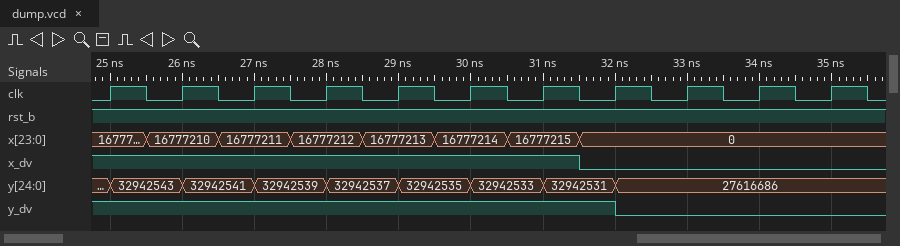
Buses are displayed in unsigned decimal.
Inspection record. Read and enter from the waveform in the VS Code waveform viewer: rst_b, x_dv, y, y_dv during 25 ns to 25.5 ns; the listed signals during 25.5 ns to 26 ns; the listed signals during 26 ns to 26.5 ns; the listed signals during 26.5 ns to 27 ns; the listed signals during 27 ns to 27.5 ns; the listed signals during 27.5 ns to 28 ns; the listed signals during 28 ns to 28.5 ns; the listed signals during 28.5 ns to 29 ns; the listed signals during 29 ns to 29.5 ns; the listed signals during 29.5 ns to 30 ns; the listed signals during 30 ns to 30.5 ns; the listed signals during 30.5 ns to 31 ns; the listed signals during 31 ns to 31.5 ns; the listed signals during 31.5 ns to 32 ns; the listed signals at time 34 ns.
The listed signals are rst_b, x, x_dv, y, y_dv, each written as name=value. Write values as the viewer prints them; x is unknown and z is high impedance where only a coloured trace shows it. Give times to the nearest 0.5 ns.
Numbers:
rst_b=1, x_dv=1, y=32942543, y_dv=1
rst_b=1, x=16777210, x_dv=1, y=32942543, y_dv=1
rst_b=1, x=16777210, x_dv=1, y=32942541, y_dv=1
rst_b=1, x=16777211, x_dv=1, y=32942541, y_dv=1
rst_b=1, x=16777211, x_dv=1, y=32942539, y_dv=1
rst_b=1, x=16777212, x_dv=1, y=32942539, y_dv=1
rst_b=1, x=16777212, x_dv=1, y=32942537, y_dv=1
rst_b=1, x=16777213, x_dv=1, y=32942537, y_dv=1
rst_b=1, x=16777213, x_dv=1, y=32942535, y_dv=1
rst_b=1, x=16777214, x_dv=1, y=32942535, y_dv=1
rst_b=1, x=16777214, x_dv=1, y=32942533, y_dv=1
rst_b=1, x=16777215, x_dv=1, y=32942533, y_dv=1
rst_b=1, x=16777215, x_dv=1, y=32942531, y_dv=1
rst_b=1, x=0, x_dv=0, y=32942531, y_dv=1
rst_b=1, x=0, x_dv=0, y=27616686, y_dv=0
